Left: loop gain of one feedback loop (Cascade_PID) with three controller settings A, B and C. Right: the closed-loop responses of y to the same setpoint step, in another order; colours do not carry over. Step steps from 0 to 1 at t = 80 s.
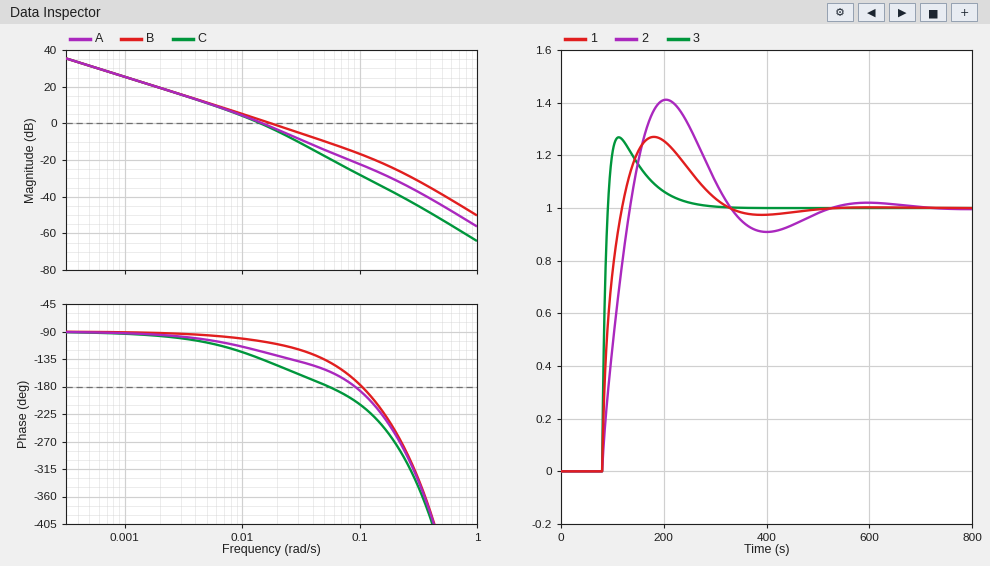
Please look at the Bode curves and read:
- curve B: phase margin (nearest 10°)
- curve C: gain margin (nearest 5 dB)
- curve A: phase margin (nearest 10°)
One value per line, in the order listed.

70°
20 dB
60°
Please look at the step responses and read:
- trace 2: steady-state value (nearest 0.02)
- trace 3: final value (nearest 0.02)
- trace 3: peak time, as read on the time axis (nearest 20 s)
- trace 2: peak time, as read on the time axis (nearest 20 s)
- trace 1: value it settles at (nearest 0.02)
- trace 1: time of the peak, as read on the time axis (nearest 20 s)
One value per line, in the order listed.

1.00
1.00
120 s
200 s
1.00
180 s
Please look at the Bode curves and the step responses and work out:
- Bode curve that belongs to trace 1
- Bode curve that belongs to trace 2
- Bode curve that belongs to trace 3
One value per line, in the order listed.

A
C
B
